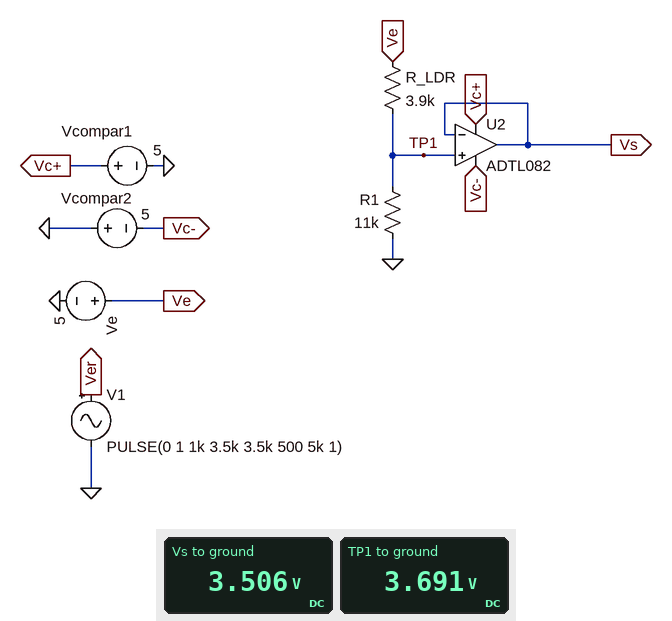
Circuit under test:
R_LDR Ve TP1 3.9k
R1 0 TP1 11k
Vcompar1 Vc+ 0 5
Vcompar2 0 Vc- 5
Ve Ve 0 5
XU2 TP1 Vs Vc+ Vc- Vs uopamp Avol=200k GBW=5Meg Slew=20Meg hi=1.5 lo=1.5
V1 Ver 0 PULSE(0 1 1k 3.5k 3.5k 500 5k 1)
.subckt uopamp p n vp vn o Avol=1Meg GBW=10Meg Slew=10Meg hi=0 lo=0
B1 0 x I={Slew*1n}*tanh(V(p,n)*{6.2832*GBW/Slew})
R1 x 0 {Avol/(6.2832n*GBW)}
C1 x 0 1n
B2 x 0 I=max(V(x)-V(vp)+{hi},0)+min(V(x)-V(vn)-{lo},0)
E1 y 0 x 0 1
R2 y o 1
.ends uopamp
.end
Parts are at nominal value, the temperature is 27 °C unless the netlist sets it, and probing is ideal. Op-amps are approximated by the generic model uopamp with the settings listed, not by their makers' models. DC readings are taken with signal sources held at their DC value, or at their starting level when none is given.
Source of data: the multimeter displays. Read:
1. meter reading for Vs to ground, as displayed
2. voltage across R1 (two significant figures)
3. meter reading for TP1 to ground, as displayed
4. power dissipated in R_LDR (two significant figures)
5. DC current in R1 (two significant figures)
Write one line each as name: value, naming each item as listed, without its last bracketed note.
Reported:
meter reading for Vs to ground, as displayed: 3.506 V
voltage across R1: 3.7 V
meter reading for TP1 to ground, as displayed: 3.691 V
power dissipated in R_LDR: 440 µW
DC current in R1: 340 µA
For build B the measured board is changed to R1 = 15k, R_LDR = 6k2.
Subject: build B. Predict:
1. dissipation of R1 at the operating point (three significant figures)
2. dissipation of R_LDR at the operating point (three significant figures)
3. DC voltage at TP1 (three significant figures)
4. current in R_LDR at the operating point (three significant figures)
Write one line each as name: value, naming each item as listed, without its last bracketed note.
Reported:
dissipation of R1 at the operating point: 834 µW
dissipation of R_LDR at the operating point: 345 µW
DC voltage at TP1: 3.54 V
current in R_LDR at the operating point: 236 µA
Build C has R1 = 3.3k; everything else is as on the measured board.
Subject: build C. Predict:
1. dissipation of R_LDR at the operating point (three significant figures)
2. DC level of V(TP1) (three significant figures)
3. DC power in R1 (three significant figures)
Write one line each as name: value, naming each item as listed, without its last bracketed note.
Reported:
dissipation of R_LDR at the operating point: 1.88 mW
DC level of V(TP1): 2.29 V
DC power in R1: 1.59 mW
